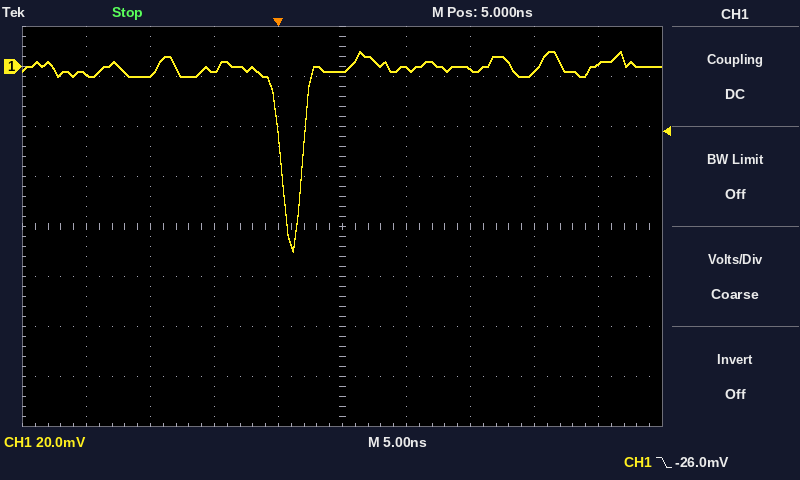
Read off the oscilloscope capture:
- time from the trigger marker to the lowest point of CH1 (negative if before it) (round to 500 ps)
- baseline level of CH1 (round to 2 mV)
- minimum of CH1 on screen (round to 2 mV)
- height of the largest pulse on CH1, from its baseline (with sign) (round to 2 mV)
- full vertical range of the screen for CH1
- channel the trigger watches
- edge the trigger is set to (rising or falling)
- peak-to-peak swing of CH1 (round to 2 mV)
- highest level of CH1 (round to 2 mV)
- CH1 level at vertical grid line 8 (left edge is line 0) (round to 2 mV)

+1.0 ns
0 mV
-74 mV
-74 mV
160 mV
CH1
falling
80 mV
6 mV
-2 mV
